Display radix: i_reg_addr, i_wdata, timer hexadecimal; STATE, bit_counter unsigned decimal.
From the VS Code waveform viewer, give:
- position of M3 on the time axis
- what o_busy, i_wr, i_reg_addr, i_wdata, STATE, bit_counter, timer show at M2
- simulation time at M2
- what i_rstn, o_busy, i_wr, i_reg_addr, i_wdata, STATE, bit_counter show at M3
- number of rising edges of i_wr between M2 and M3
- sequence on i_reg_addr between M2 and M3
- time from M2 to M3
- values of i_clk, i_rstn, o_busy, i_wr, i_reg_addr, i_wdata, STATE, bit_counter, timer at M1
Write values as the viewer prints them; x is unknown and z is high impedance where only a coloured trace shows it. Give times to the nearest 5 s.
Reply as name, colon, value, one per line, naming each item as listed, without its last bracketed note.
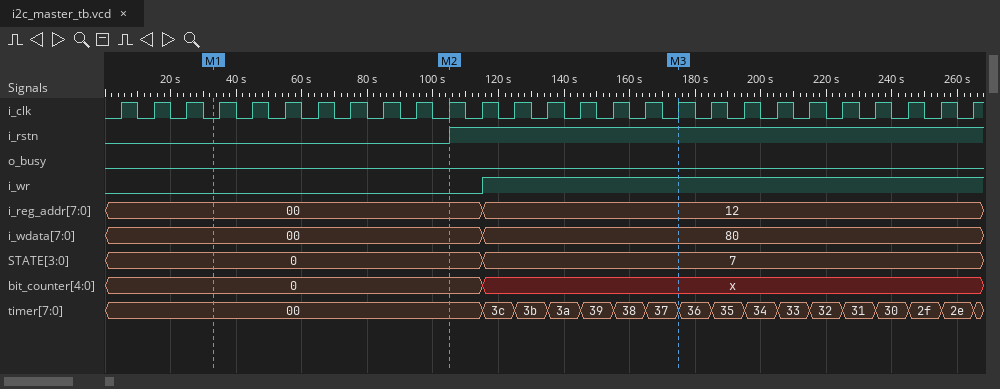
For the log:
position of M3 on the time axis: 175 s
what o_busy, i_wr, i_reg_addr, i_wdata, STATE, bit_counter, timer show at M2: o_busy=0, i_wr=0, i_reg_addr=00, i_wdata=00, STATE=0, bit_counter=0, timer=00
simulation time at M2: 105 s
what i_rstn, o_busy, i_wr, i_reg_addr, i_wdata, STATE, bit_counter show at M3: i_rstn=1, o_busy=0, i_wr=1, i_reg_addr=12, i_wdata=80, STATE=7, bit_counter=x
number of rising edges of i_wr between M2 and M3: 1
sequence on i_reg_addr between M2 and M3: 00, 12
time from M2 to M3: 70 s
values of i_clk, i_rstn, o_busy, i_wr, i_reg_addr, i_wdata, STATE, bit_counter, timer at M1: i_clk=0, i_rstn=0, o_busy=0, i_wr=0, i_reg_addr=00, i_wdata=00, STATE=0, bit_counter=0, timer=00
